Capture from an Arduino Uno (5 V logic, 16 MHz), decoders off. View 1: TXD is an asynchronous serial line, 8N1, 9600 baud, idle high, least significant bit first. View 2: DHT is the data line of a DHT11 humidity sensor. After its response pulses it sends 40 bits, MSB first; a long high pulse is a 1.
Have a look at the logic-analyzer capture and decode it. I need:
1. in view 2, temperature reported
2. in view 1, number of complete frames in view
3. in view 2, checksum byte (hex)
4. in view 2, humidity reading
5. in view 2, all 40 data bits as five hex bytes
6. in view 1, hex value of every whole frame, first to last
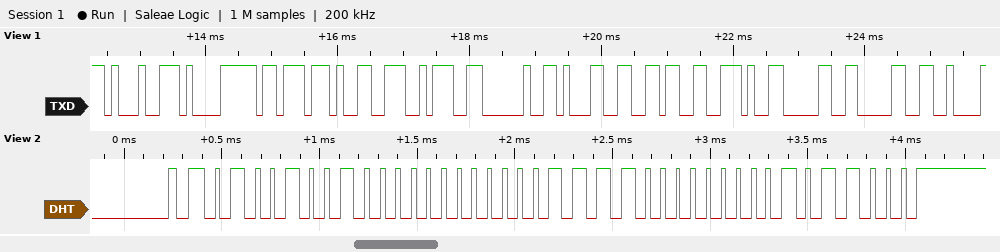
15.0 °C
11
0x58
73 %
49 00 0F 00 58
0x91 0xE1 0xBB 0x99 0x3A 0x20 0x31 0x36 0x2E 0x30 0x30
